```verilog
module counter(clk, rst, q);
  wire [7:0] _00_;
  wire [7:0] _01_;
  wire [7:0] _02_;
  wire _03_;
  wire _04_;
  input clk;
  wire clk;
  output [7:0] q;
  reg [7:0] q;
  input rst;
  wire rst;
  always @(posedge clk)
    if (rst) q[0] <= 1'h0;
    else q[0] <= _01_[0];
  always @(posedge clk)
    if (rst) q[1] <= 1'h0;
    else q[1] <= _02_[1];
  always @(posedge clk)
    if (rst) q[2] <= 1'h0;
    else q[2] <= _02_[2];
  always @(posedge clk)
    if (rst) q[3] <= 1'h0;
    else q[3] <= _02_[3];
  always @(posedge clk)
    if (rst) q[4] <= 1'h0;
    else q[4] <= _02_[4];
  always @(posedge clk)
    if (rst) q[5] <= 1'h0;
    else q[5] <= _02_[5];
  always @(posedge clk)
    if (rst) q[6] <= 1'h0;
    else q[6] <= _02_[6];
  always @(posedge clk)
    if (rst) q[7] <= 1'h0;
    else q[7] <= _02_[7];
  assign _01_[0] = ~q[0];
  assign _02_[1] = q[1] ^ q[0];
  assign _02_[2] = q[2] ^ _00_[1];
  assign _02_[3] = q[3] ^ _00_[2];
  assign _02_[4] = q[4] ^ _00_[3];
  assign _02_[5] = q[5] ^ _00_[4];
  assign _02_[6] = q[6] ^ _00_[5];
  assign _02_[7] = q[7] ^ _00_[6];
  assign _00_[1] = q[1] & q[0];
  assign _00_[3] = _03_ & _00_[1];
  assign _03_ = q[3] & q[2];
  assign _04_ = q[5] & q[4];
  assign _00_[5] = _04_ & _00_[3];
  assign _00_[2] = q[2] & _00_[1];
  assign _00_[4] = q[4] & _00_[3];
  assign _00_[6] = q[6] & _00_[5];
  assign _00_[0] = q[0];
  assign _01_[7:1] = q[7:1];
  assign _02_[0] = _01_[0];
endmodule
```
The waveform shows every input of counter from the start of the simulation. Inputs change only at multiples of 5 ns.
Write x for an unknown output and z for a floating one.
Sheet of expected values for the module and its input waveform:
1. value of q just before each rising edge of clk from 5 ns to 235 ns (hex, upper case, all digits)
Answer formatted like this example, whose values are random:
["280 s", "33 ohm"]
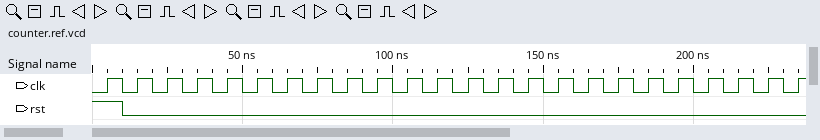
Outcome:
["x, 00, 01, 02, 03, 04, 05, 06, 07, 08, 09, 0A, 0B, 0C, 0D, 0E, 0F, 10, 11, 12, 13, 14, 15, 16"]
